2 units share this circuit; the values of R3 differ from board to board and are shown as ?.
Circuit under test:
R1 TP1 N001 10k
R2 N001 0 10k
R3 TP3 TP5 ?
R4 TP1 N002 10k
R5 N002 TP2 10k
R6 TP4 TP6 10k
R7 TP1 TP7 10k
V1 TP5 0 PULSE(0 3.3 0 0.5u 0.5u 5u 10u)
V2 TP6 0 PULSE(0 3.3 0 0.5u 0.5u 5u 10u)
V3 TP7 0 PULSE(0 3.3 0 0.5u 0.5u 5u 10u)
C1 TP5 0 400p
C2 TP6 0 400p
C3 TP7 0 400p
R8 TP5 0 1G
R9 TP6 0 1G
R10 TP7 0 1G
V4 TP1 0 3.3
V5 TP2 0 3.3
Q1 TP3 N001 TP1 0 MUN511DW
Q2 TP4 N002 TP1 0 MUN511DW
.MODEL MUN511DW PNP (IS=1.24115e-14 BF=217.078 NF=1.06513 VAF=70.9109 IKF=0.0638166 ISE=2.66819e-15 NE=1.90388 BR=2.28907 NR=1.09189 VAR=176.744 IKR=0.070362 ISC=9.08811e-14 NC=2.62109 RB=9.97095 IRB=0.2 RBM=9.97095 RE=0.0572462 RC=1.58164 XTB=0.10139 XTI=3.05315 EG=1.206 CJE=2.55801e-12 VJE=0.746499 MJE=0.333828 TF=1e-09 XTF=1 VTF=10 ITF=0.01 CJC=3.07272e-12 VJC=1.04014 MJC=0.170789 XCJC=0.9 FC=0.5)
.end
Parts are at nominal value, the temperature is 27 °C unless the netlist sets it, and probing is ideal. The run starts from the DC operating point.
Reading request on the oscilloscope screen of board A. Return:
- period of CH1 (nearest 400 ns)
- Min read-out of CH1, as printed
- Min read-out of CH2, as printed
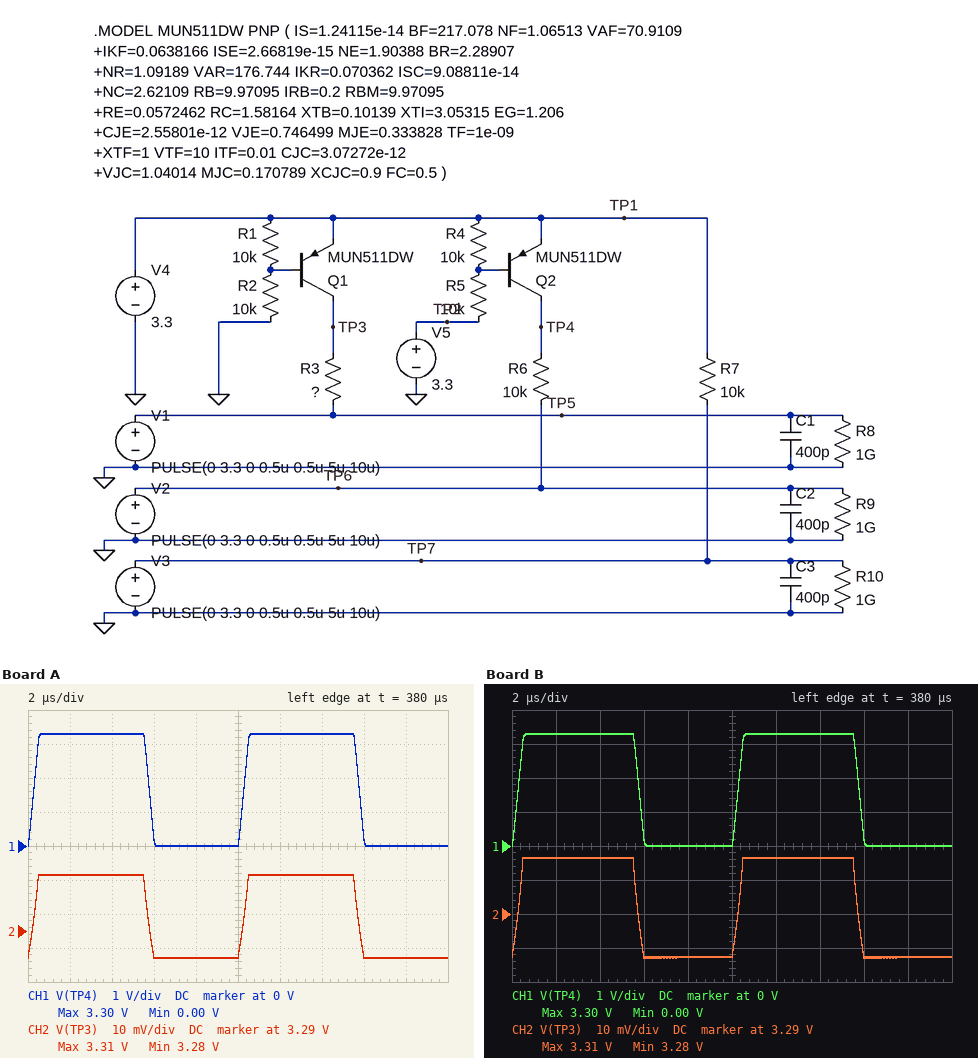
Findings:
10.0 µs
0.00 V
3.28 V
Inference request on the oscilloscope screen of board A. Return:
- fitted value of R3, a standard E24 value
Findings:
4.3 kΩ
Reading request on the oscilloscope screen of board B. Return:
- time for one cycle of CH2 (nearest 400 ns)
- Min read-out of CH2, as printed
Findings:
10.0 µs
3.28 V
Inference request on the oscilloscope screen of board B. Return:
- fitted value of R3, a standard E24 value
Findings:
3.3 kΩ
